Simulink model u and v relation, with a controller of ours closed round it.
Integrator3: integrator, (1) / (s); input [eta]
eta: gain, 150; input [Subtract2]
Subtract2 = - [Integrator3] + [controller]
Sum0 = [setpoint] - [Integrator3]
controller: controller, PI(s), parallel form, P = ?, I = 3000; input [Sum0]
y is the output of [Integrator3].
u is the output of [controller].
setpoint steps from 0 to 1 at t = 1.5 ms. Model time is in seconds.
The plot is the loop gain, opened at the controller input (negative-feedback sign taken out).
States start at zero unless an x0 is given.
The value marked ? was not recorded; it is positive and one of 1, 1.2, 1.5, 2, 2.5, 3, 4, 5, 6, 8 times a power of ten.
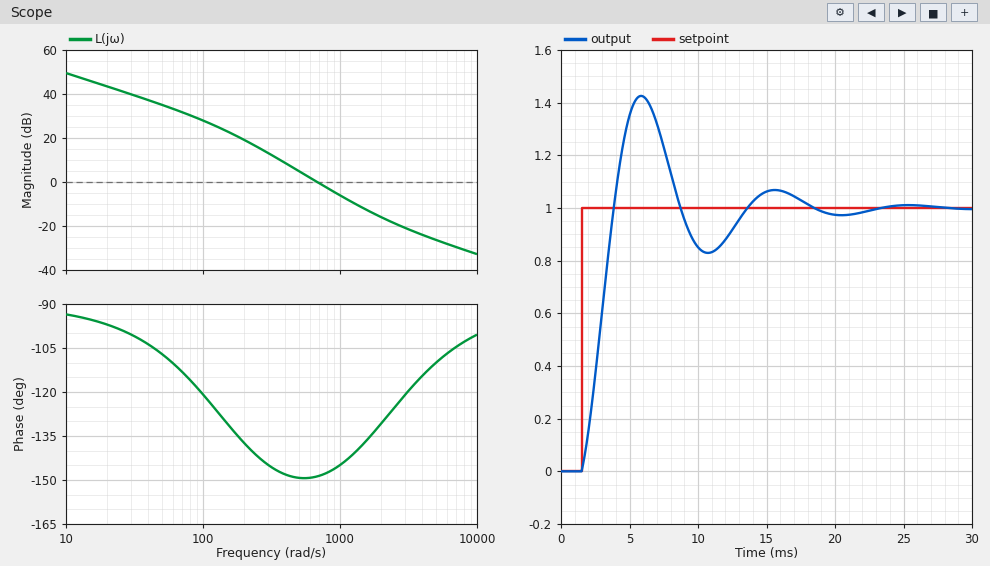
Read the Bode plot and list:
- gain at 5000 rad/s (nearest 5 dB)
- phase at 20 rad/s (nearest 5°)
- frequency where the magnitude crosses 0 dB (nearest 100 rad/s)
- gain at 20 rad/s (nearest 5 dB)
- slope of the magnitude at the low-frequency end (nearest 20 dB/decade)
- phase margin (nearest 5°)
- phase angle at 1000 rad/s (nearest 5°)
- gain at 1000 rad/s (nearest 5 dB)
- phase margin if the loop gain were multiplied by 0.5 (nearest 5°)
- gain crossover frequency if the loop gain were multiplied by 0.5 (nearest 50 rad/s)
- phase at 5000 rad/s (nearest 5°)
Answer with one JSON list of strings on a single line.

["-25 dB", "-95°", "700 rad/s", "45 dB", "-20 dB/decade", "30°", "-145°", "-5 dB", "30°", "450 rad/s", "-110°"]
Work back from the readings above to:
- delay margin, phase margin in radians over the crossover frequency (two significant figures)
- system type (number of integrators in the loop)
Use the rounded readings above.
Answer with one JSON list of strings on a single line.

["0.00075 s", "1"]
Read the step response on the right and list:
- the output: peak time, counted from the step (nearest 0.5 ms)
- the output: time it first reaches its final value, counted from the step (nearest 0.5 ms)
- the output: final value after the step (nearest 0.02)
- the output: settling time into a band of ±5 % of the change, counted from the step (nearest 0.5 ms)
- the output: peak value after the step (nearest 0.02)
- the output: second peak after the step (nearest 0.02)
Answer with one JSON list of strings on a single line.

["4.5 ms", "2.5 ms", "1.00", "15.5 ms", "1.42", "1.06"]
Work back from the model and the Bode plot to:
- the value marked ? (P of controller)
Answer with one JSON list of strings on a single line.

["1.5"]
